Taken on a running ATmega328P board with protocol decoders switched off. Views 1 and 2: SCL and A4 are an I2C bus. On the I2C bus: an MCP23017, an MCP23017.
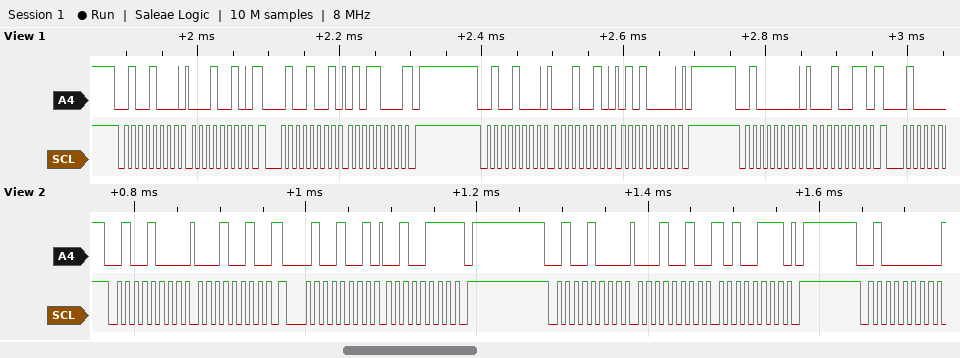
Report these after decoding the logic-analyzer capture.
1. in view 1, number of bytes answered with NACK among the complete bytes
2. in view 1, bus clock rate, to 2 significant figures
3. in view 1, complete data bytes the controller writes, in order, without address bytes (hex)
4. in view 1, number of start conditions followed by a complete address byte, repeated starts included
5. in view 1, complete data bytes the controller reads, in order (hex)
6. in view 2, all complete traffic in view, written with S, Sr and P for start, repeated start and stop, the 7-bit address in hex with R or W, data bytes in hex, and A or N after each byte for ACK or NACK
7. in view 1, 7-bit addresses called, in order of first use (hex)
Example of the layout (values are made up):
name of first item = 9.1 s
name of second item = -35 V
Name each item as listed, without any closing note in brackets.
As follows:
in view 1, number of bytes answered with NACK among the complete bytes = 1
in view 1, bus clock rate, to 2 significant figures = 100 kHz
in view 1, complete data bytes the controller writes, in order, without address bytes = 12 12 50 13
in view 1, number of start conditions followed by a complete address byte, repeated starts included = 4
in view 1, complete data bytes the controller reads, in order = 58
in view 2, all complete traffic in view, written with S, Sr and P for start, repeated start and stop, the 7-bit address in hex with R or W, data bytes in hex, and A or N after each byte for ACK or NACK = S 24W A 12 A Sr 24R A 27 N P S 24W A 12 A A7 A P S 20W A
in view 1, 7-bit addresses called, in order of first use = 0x24 0x20
